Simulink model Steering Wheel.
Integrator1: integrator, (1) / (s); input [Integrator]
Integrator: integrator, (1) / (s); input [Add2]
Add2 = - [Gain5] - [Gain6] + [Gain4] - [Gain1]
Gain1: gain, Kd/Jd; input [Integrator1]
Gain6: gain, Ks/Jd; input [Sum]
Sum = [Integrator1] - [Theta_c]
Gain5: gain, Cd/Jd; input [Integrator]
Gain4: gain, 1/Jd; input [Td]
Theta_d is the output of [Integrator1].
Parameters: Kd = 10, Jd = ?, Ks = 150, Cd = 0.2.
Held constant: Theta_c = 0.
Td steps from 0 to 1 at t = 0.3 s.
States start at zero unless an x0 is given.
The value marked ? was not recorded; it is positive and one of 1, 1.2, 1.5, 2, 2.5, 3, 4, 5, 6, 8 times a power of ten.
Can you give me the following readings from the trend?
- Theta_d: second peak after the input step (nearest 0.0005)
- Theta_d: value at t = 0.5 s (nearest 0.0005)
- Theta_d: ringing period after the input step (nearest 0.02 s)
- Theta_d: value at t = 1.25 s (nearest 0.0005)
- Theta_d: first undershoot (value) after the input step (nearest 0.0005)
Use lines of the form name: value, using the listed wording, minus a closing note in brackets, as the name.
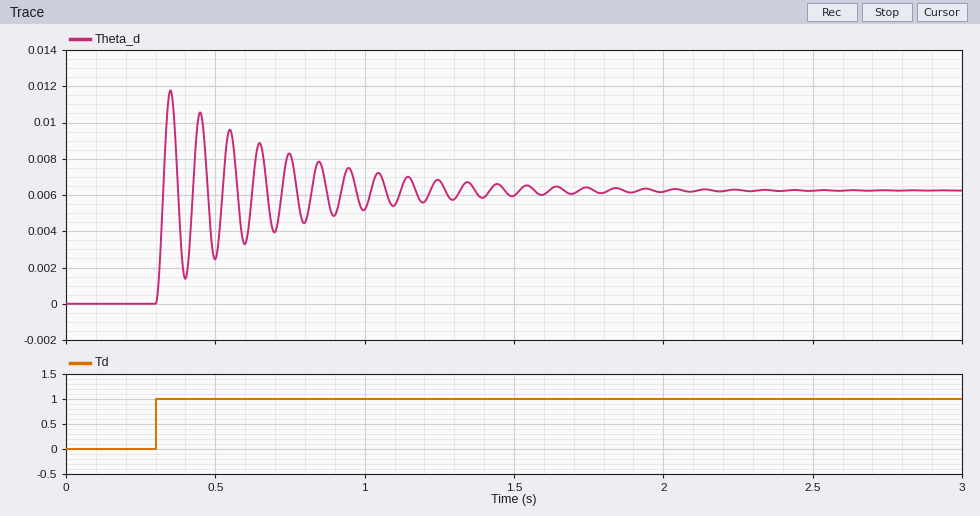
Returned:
Theta_d: second peak after the input step: 0.0105
Theta_d: value at t = 0.5 s: 0.0025
Theta_d: ringing period after the input step: 0.10 s
Theta_d: value at t = 1.25 s: 0.0070
Theta_d: first undershoot (value) after the input step: 0.0015
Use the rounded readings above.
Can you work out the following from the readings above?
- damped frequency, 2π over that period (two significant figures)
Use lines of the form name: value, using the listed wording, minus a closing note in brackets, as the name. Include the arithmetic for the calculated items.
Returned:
damped frequency, 2π over that period: 2π / 0.1 = 63 rad/s
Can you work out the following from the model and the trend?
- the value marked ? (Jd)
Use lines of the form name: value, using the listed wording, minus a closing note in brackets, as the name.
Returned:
the value marked ?: 0.04
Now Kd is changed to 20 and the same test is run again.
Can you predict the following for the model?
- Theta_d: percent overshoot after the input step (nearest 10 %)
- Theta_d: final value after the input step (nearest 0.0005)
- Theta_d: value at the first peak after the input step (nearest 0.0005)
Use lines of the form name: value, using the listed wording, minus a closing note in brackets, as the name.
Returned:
Theta_d: percent overshoot after the input step: 90 %
Theta_d: final value after the input step: 0.0060
Theta_d: value at the first peak after the input step: 0.0110
